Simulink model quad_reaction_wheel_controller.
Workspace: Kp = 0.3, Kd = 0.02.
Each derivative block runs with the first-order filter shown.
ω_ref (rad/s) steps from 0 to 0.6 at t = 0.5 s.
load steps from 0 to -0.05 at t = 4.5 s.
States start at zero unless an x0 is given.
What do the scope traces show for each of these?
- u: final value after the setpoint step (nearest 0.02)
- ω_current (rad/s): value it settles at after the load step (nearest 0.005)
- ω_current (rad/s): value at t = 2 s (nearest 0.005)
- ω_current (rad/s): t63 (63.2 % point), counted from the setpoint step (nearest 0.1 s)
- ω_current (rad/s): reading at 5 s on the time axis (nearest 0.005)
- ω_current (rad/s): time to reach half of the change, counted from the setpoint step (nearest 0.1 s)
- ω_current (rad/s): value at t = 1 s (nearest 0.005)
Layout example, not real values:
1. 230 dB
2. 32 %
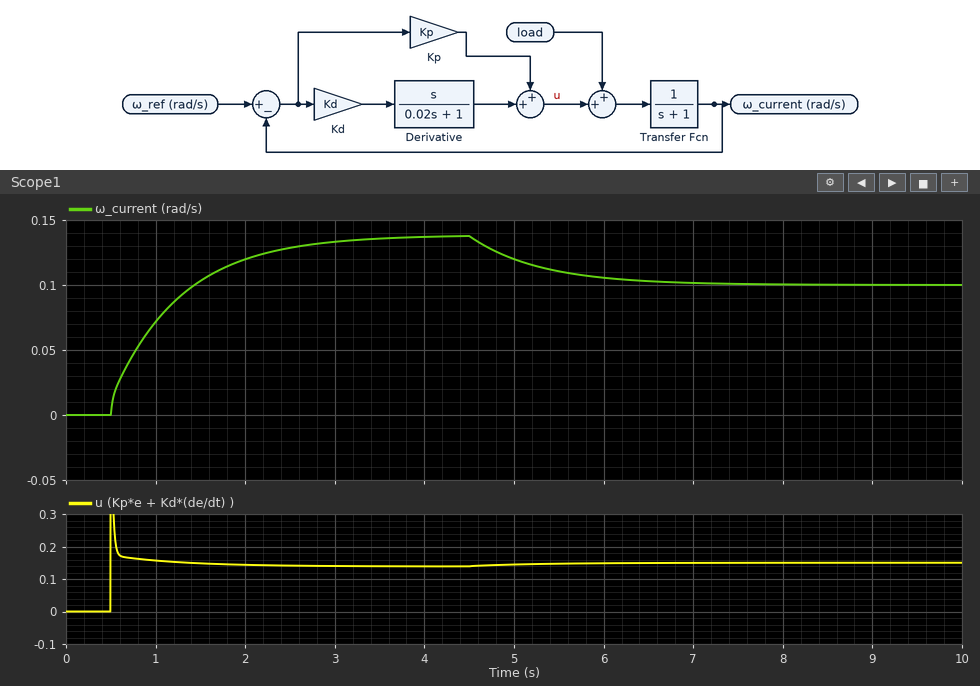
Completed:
1. 0.14
2. 0.100
3. 0.120
4. 0.7 s
5. 0.120
6. 0.5 s
7. 0.070
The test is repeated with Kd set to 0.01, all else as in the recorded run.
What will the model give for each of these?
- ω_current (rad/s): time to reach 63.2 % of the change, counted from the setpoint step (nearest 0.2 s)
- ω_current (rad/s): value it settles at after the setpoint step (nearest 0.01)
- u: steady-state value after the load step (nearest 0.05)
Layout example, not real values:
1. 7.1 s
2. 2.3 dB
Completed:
1. 0.8 s
2. 0.14
3. 0.15
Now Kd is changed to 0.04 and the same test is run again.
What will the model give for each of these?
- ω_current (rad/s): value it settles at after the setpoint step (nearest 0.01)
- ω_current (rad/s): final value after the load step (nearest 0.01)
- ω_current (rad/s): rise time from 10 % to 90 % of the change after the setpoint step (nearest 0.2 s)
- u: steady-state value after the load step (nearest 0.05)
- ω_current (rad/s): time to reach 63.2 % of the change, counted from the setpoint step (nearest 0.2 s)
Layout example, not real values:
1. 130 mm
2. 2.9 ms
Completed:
1. 0.14
2. 0.10
3. 1.6 s
4. 0.15
5. 0.6 s
